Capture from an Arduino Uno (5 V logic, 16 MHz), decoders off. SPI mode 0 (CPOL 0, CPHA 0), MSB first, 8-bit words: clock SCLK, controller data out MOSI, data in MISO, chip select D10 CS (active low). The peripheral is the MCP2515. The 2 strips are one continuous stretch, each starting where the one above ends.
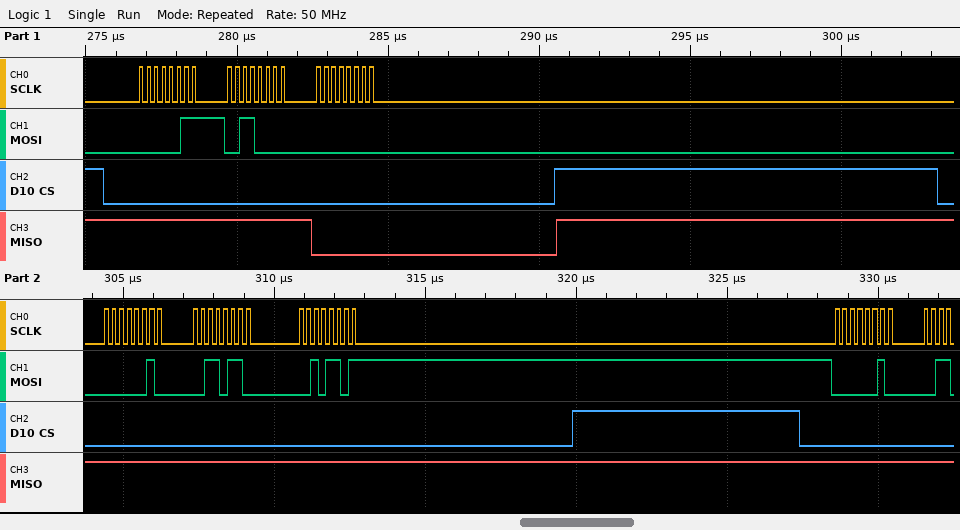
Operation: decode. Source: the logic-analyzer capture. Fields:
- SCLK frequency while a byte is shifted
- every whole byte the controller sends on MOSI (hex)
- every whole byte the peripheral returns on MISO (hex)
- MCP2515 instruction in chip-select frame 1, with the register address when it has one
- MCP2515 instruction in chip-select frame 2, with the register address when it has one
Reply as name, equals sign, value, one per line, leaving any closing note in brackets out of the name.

SCLK frequency while a byte is shifted = 4 MHz
every whole byte the controller sends on MOSI = 03 30 00 02 36 2D 02
every whole byte the peripheral returns on MISO = FF FF 00 FF FF FF FF
MCP2515 instruction in chip-select frame 1, with the register address when it has one = READ 0x30
MCP2515 instruction in chip-select frame 2, with the register address when it has one = WRITE 0x36
